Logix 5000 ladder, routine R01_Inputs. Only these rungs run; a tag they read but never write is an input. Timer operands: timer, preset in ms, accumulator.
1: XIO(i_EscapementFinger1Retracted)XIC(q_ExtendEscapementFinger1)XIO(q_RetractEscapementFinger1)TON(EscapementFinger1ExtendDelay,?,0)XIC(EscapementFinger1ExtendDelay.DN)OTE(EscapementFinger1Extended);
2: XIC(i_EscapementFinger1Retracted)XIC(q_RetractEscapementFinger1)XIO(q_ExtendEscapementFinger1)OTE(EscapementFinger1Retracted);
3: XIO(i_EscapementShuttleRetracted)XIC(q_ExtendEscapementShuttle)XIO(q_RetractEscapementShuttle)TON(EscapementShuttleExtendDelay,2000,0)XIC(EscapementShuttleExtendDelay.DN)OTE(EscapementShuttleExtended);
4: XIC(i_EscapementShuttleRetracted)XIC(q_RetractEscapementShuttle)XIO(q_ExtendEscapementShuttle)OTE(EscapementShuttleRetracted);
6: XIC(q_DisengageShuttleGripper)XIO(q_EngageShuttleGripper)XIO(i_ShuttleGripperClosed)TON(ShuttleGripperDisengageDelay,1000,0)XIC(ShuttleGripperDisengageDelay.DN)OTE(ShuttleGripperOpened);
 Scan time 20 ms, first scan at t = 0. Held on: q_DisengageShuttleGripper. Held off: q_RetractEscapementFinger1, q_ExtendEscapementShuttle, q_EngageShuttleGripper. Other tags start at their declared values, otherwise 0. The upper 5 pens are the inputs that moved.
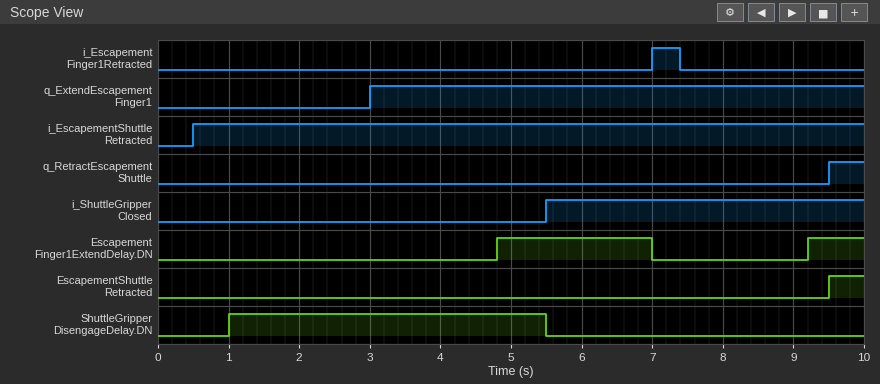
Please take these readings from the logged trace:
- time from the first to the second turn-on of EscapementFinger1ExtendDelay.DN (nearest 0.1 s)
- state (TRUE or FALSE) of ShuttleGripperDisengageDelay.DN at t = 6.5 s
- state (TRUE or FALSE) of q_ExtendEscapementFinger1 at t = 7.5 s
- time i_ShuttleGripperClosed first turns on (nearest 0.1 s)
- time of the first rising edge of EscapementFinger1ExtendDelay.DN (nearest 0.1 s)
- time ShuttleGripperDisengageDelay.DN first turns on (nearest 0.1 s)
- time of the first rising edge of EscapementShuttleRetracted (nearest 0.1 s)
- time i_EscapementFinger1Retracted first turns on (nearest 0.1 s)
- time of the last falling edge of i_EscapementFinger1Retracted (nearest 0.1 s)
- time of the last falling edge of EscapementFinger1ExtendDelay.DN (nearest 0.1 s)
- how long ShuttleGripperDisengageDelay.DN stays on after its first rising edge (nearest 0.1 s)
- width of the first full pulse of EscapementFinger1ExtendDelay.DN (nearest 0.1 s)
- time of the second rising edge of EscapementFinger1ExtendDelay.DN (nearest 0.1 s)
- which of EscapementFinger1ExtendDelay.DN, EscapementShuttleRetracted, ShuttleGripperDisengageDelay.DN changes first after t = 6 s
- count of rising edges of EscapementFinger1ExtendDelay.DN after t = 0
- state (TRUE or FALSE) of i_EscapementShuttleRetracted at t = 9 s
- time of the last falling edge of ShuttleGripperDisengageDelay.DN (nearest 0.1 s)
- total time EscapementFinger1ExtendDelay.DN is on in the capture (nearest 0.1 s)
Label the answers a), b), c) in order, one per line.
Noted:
a) 4.4 s
b) FALSE
c) TRUE
d) 5.5 s
e) 4.8 s
f) 1.0 s
g) 9.5 s
h) 7.0 s
i) 7.4 s
j) 7.0 s
k) 4.5 s
l) 2.2 s
m) 9.2 s
n) EscapementFinger1ExtendDelay.DN
o) 2
p) TRUE
q) 5.5 s
r) 3.0 s
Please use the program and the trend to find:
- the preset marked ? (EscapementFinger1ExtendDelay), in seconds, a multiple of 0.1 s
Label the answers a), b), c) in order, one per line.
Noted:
a) 1.8 s
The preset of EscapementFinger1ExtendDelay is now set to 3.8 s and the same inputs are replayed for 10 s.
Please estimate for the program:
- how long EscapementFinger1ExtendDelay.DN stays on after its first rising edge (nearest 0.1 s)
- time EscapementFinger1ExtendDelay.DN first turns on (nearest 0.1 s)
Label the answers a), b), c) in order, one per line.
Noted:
a) 0.2 s
b) 6.8 s
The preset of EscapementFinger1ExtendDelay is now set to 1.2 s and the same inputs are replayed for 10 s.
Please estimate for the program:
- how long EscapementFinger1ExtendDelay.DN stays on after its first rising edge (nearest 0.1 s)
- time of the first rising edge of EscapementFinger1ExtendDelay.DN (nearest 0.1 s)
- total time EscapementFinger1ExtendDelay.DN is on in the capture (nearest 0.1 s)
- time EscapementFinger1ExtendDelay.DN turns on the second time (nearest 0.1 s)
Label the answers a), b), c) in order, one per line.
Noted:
a) 2.8 s
b) 4.2 s
c) 4.2 s
d) 8.6 s
